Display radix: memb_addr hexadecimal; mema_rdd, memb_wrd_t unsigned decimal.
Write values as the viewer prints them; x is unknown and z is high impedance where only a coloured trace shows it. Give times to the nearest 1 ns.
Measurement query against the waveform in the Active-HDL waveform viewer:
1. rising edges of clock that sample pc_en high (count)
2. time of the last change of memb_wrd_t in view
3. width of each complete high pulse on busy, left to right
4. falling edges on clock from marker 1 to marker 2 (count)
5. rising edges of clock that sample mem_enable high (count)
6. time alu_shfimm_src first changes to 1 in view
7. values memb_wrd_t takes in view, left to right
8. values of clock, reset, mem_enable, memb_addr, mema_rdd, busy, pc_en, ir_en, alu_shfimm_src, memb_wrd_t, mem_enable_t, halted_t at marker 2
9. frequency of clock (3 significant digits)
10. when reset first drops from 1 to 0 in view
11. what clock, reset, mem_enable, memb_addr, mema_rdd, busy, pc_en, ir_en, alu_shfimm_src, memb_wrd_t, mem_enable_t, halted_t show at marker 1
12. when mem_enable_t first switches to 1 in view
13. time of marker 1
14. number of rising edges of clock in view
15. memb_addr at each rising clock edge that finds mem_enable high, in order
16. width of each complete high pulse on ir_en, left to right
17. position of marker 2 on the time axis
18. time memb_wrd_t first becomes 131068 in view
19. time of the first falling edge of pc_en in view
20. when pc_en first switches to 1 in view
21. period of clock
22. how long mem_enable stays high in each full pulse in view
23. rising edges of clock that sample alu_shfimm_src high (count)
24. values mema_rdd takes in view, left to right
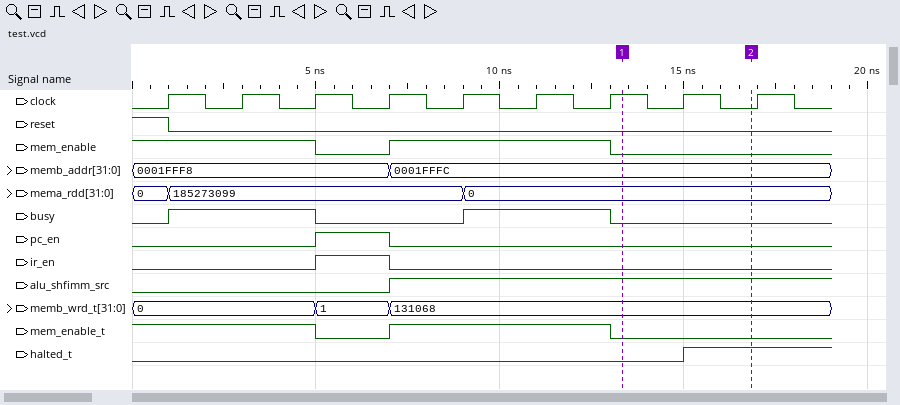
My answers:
1
7 ns
4 ns, 4 ns
2
6
7 ns
0, 1, 131068
clock=0, reset=0, mem_enable=0, memb_addr=0001FFFC, mema_rdd=0, busy=0, pc_en=0, ir_en=0, alu_shfimm_src=1, memb_wrd_t=131068, mem_enable_t=0, halted_t=1
500 MHz
1 ns
clock=1, reset=0, mem_enable=0, memb_addr=0001FFFC, mema_rdd=0, busy=0, pc_en=0, ir_en=0, alu_shfimm_src=1, memb_wrd_t=131068, mem_enable_t=0, halted_t=0
7 ns
13 ns
9
0001FFF8, 0001FFF8, 0001FFF8, 0001FFFC, 0001FFFC, 0001FFFC
2 ns
17 ns
7 ns
7 ns
5 ns
2 ns
6 ns
5
0, 185273099, 0
